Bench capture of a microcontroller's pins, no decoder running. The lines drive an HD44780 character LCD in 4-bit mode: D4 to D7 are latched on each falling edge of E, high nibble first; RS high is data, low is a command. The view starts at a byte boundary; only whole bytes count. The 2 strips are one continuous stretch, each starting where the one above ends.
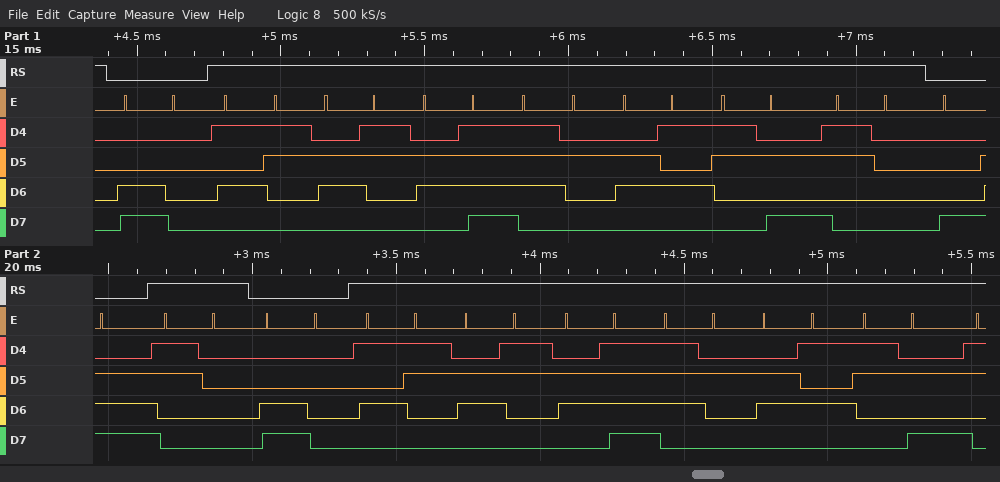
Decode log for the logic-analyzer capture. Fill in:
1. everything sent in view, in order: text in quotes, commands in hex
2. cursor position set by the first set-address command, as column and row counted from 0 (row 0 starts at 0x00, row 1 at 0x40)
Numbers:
0xC0 "Score:0" 0x8E "0" 0xC0 "Score:"
column 0, row 1
